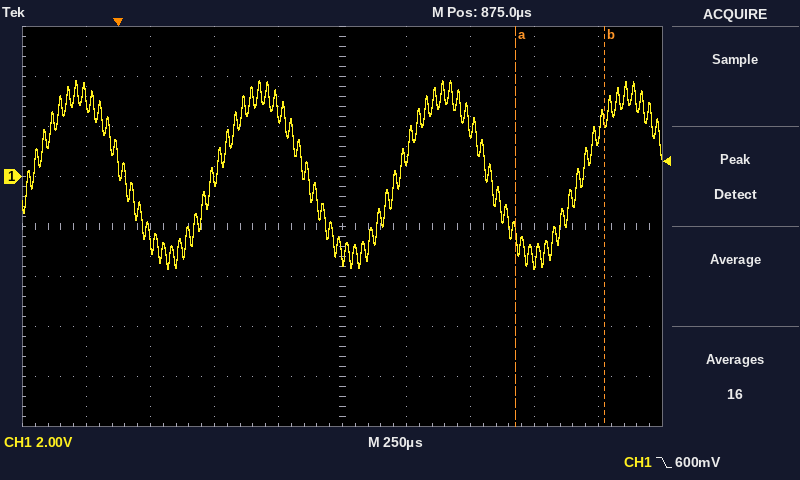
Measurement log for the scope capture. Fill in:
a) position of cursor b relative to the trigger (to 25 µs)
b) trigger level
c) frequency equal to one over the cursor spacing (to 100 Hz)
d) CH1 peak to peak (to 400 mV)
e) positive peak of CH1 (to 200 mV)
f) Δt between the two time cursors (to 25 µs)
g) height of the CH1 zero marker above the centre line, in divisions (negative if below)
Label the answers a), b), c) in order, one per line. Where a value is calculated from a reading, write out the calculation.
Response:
a) +1.900 ms
b) 600 mV
c) 1 / 350 µs ≈ 2.9 kHz
d) 7.6 V
e) 3.8 V
f) 350 µs
g) +1.0 div
